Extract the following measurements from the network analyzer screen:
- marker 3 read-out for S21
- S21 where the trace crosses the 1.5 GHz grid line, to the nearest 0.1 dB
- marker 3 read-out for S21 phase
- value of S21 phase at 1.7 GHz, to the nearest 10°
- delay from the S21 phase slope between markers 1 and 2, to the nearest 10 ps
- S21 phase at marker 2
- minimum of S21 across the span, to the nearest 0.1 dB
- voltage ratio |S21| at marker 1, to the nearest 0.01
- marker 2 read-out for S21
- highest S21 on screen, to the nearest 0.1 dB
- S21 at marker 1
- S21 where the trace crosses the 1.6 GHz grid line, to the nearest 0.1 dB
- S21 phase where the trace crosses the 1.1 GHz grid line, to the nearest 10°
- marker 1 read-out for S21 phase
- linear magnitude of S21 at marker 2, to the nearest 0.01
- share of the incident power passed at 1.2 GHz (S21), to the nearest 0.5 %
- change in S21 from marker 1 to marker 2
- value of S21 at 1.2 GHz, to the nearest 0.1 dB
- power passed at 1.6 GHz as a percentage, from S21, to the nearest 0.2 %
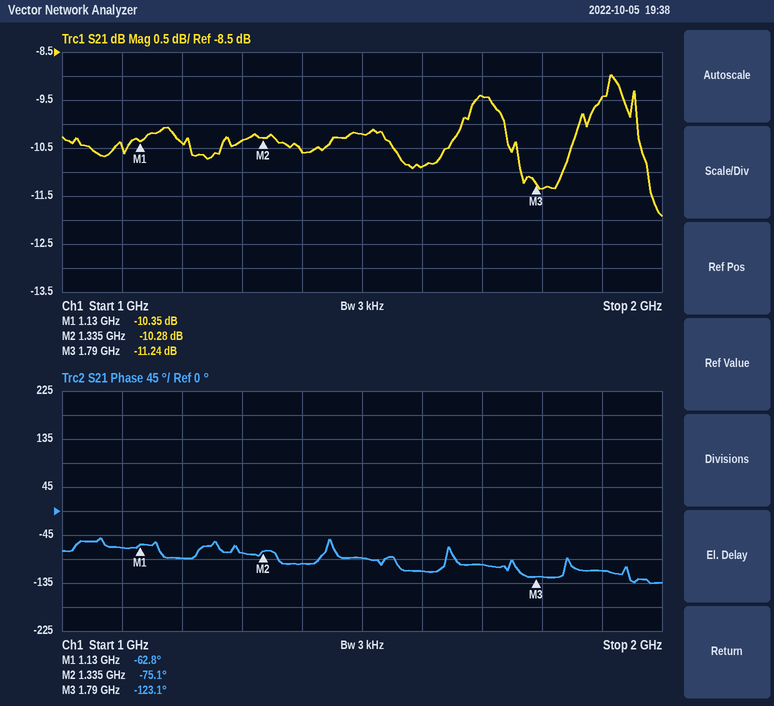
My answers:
-11.24 dB
-10.2 dB
-123.1°
-100°
170 ps
-75.1°
-11.9 dB
0.30
-10.28 dB
-9.0 dB
-10.35 dB
-10.9 dB
-70°
-62.8°
0.31
9.0 %
0.07 dB
-10.4 dB
8.2 %
